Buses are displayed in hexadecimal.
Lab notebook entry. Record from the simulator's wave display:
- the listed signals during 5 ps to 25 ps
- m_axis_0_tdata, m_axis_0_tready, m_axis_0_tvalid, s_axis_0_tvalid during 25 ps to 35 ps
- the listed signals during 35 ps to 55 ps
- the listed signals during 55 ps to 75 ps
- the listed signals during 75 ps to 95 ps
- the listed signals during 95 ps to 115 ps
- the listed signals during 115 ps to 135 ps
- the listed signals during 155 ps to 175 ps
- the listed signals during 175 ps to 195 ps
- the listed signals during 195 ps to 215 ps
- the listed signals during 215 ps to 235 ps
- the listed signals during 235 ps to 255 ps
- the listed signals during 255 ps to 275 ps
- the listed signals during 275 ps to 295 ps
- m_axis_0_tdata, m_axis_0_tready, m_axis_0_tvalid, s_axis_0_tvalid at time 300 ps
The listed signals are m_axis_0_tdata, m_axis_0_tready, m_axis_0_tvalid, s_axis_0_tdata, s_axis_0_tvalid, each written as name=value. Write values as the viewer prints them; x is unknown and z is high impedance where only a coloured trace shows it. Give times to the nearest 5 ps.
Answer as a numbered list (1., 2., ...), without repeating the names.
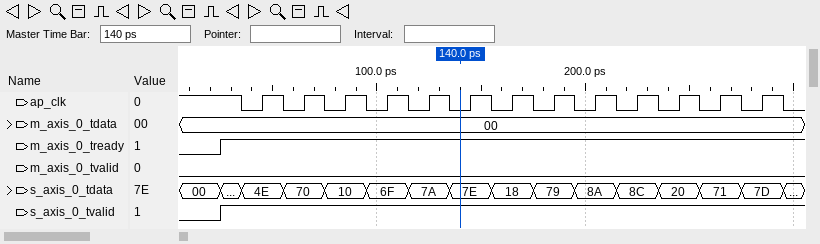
1. m_axis_0_tdata=00, m_axis_0_tready=0, m_axis_0_tvalid=0, s_axis_0_tdata=00, s_axis_0_tvalid=0
2. m_axis_0_tdata=00, m_axis_0_tready=1, m_axis_0_tvalid=0, s_axis_0_tvalid=1
3. m_axis_0_tdata=00, m_axis_0_tready=1, m_axis_0_tvalid=0, s_axis_0_tdata=4E, s_axis_0_tvalid=1
4. m_axis_0_tdata=00, m_axis_0_tready=1, m_axis_0_tvalid=0, s_axis_0_tdata=70, s_axis_0_tvalid=1
5. m_axis_0_tdata=00, m_axis_0_tready=1, m_axis_0_tvalid=0, s_axis_0_tdata=10, s_axis_0_tvalid=1
6. m_axis_0_tdata=00, m_axis_0_tready=1, m_axis_0_tvalid=0, s_axis_0_tdata=6F, s_axis_0_tvalid=1
7. m_axis_0_tdata=00, m_axis_0_tready=1, m_axis_0_tvalid=0, s_axis_0_tdata=7A, s_axis_0_tvalid=1
8. m_axis_0_tdata=00, m_axis_0_tready=1, m_axis_0_tvalid=0, s_axis_0_tdata=18, s_axis_0_tvalid=1
9. m_axis_0_tdata=00, m_axis_0_tready=1, m_axis_0_tvalid=0, s_axis_0_tdata=79, s_axis_0_tvalid=1
10. m_axis_0_tdata=00, m_axis_0_tready=1, m_axis_0_tvalid=0, s_axis_0_tdata=8A, s_axis_0_tvalid=1
11. m_axis_0_tdata=00, m_axis_0_tready=1, m_axis_0_tvalid=0, s_axis_0_tdata=8C, s_axis_0_tvalid=1
12. m_axis_0_tdata=00, m_axis_0_tready=1, m_axis_0_tvalid=0, s_axis_0_tdata=20, s_axis_0_tvalid=1
13. m_axis_0_tdata=00, m_axis_0_tready=1, m_axis_0_tvalid=0, s_axis_0_tdata=71, s_axis_0_tvalid=1
14. m_axis_0_tdata=00, m_axis_0_tready=1, m_axis_0_tvalid=0, s_axis_0_tdata=7D, s_axis_0_tvalid=1
15. m_axis_0_tdata=00, m_axis_0_tready=1, m_axis_0_tvalid=0, s_axis_0_tvalid=1
